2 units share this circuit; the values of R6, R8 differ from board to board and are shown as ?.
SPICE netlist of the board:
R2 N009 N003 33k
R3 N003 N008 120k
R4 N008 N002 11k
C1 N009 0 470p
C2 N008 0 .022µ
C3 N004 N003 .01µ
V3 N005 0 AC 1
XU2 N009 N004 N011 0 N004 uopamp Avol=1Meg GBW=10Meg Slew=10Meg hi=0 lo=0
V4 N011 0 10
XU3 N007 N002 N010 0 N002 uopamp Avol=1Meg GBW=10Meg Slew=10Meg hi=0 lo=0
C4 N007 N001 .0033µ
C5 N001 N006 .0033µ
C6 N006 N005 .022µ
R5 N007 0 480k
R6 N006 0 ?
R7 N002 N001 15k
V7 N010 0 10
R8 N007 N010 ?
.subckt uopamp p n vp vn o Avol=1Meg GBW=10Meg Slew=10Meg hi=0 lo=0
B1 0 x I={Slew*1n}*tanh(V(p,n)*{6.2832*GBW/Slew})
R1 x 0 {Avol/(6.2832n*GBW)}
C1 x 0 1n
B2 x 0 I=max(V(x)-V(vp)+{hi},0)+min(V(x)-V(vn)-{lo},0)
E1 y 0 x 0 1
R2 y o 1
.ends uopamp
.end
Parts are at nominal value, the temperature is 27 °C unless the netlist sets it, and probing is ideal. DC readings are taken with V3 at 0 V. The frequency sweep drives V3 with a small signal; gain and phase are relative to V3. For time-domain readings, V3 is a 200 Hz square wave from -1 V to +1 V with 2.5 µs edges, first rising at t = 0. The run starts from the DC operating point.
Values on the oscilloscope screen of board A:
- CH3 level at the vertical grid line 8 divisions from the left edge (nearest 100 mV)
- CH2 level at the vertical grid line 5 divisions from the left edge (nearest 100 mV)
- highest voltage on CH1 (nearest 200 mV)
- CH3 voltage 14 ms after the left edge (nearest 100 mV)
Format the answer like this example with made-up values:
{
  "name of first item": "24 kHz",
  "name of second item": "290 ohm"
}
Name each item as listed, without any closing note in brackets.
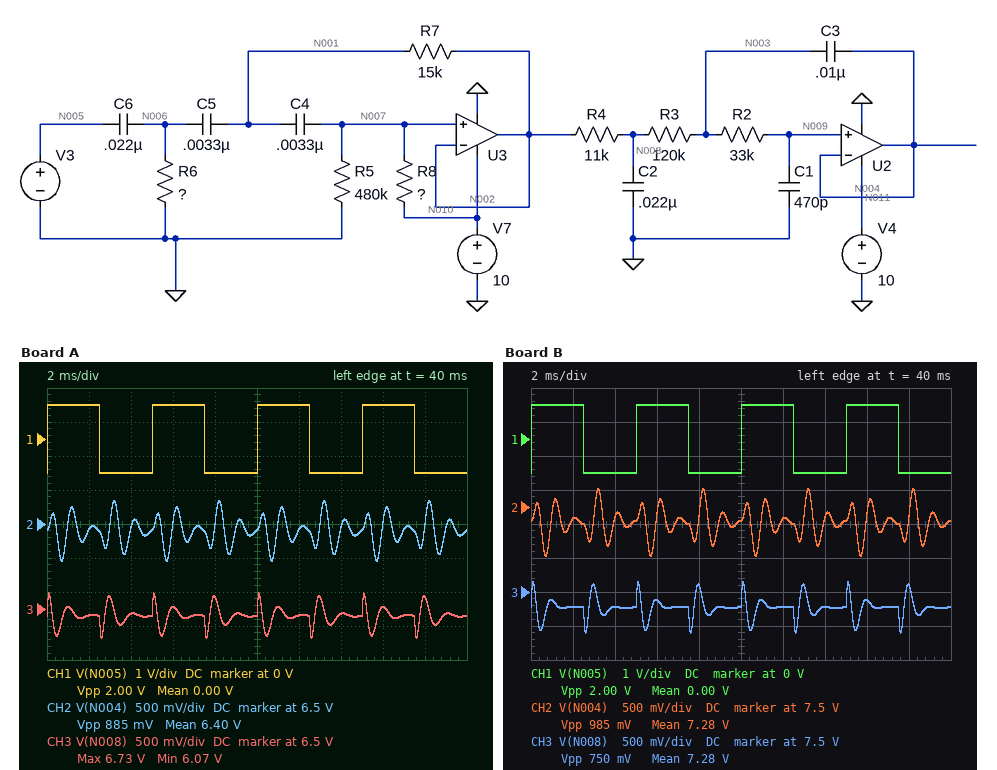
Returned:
{
  "CH3 level at the vertical grid line 8 divisions from the left edge": "6.5 V",
  "CH2 level at the vertical grid line 5 divisions from the left edge": "6.4 V",
  "highest voltage on CH1": "1.0 V",
  "CH3 voltage 14 ms after the left edge": "6.4 V"
}
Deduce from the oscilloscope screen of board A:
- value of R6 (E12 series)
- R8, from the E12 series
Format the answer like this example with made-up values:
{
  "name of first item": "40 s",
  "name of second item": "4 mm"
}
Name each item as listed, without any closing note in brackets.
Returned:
{
  "value of R6": "5.6 kΩ",
  "R8, from the E12 series": "270 kΩ"
}
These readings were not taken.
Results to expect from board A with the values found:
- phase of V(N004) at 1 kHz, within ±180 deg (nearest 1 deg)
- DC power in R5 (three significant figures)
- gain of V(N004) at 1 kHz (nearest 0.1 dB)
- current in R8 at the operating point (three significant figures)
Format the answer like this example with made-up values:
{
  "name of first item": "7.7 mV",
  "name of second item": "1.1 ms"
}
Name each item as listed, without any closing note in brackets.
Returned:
{
  "phase of V(N004) at 1 kHz, within ±180 deg": "17 deg",
  "DC power in R5": "85.3 µW",
  "gain of V(N004) at 1 kHz": "-0.5 dB",
  "current in R8 at the operating point": "13.3 µA"
}
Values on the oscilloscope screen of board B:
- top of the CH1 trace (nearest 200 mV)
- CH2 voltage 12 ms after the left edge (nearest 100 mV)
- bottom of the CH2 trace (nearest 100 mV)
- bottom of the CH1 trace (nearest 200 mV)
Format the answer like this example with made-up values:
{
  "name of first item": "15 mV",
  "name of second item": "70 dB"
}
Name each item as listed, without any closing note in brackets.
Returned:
{
  "top of the CH1 trace": "1.0 V",
  "CH2 voltage 12 ms after the left edge": "7.3 V",
  "bottom of the CH2 trace": "6.8 V",
  "bottom of the CH1 trace": "-1.0 V"
}
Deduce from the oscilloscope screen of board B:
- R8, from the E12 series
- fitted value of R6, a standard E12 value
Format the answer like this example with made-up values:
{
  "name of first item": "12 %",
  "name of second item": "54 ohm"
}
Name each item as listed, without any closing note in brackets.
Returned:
{
  "R8, from the E12 series": "180 kΩ",
  "fitted value of R6, a standard E12 value": "12 kΩ"
}
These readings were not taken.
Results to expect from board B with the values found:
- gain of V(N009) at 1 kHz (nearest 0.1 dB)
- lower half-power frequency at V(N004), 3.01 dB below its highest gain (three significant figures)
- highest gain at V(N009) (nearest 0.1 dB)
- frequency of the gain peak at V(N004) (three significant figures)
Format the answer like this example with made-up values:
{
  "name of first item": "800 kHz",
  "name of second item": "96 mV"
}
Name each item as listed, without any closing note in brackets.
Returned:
{
  "gain of V(N009) at 1 kHz": "-0.6 dB",
  "lower half-power frequency at V(N004), 3.01 dB below its highest gain": "909 Hz",
  "highest gain at V(N009)": "0.5 dB",
  "frequency of the gain peak at V(N004)": "1.13 kHz"
}
